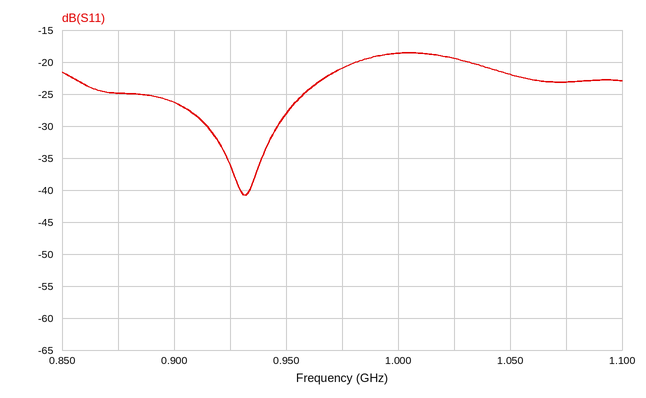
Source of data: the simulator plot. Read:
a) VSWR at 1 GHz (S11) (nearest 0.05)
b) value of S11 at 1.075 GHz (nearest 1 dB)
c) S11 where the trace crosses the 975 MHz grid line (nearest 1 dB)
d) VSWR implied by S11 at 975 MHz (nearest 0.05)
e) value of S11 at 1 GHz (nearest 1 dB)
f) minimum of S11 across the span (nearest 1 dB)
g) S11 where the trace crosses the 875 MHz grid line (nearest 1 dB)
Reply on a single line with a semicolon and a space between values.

1.25; -23 dB; -21 dB; 1.20; -19 dB; -41 dB; -25 dB
